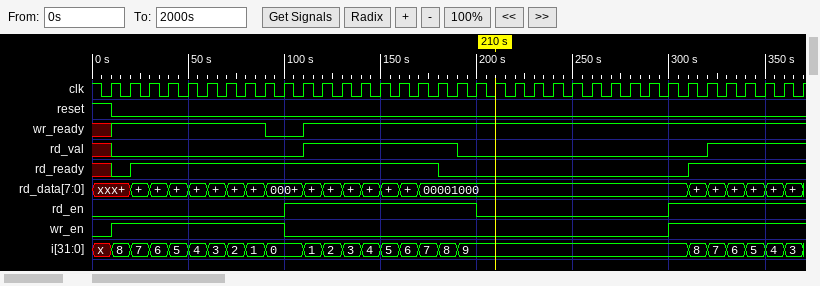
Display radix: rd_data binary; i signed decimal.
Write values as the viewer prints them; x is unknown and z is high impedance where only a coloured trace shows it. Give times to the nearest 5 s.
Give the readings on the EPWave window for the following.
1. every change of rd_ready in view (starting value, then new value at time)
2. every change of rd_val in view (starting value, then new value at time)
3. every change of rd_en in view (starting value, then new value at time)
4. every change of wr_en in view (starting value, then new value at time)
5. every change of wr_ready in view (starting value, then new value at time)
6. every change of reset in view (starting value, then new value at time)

x, 0 at 10 s, 1 at 20 s, 0 at 180 s, 1 at 310 s
x, 0 at 10 s, 1 at 110 s, 0 at 190 s, 1 at 320 s
0, 1 at 100 s, 0 at 200 s, 1 at 300 s
0, 1 at 10 s, 0 at 100 s, 1 at 300 s
x, 1 at 10 s, 0 at 90 s, 1 at 110 s
1, 0 at 10 s
